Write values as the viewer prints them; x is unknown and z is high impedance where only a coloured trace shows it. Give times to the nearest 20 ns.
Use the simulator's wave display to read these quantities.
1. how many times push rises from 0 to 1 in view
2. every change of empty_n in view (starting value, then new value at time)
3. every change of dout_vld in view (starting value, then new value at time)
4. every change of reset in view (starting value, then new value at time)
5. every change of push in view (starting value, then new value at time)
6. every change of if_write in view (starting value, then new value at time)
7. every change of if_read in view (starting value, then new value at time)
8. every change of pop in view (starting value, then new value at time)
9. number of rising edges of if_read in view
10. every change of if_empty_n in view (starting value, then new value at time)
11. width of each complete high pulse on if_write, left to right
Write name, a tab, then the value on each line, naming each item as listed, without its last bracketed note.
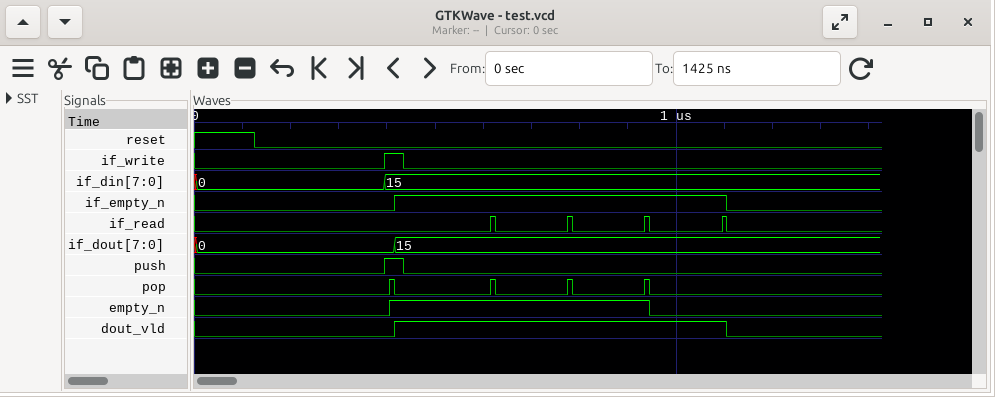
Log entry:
how many times push rises from 0 to 1 in view	1
every change of empty_n in view	0, 1 at 400 ns, 0 at 940 ns
every change of dout_vld in view	0, 1 at 420 ns, 0 at 1100 ns
every change of reset in view	1, 0 at 120 ns
every change of push in view	0, 1 at 400 ns, 0 at 440 ns
every change of if_write in view	0, 1 at 400 ns, 0 at 440 ns
every change of if_read in view	0, 1 at 620 ns, 0 at 620 ns, 1 at 780 ns, 0 at 780 ns, 1 at 940 ns, 0 at 940 ns, 1 at 1100 ns, 0 at 1100 ns
every change of pop in view	0, 1 at 400 ns, 0 at 420 ns, 1 at 620 ns, 0 at 620 ns, 1 at 780 ns, 0 at 780 ns, 1 at 940 ns, 0 at 940 ns
number of rising edges of if_read in view	4
every change of if_empty_n in view	0, 1 at 420 ns, 0 at 1100 ns
width of each complete high pulse on if_write, left to right	40 ns
